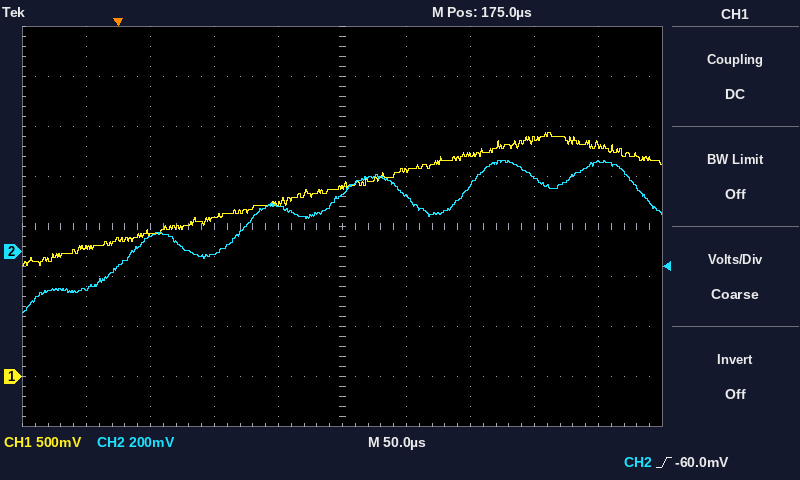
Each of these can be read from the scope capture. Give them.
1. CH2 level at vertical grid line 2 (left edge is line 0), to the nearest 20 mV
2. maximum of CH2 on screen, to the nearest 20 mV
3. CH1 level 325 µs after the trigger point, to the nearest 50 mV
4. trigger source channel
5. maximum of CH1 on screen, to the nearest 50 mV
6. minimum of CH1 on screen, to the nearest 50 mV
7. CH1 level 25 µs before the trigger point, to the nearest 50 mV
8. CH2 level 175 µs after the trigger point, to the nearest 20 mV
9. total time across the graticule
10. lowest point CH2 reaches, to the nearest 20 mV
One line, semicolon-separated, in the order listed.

60 mV; 360 mV; 2.35 V; CH2; 2.45 V; 1.10 V; 1.30 V; 220 mV; 500 µs; -240 mV
